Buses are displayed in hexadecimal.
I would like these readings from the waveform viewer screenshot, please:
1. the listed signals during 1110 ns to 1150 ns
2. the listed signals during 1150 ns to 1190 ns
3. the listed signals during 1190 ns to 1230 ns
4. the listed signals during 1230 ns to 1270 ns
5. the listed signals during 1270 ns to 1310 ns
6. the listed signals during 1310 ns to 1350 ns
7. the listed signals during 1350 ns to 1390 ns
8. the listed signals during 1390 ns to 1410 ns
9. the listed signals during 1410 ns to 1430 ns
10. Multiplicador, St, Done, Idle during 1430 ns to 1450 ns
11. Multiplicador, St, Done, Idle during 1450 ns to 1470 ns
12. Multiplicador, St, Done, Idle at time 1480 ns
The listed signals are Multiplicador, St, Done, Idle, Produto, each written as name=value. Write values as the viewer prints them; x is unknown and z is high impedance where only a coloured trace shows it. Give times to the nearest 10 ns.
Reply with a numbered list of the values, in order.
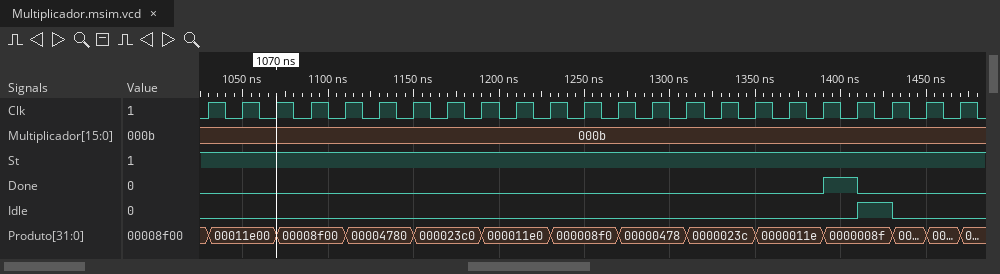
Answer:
1. Multiplicador=000b, St=1, Done=0, Idle=0, Produto=00004780
2. Multiplicador=000b, St=1, Done=0, Idle=0, Produto=000023c0
3. Multiplicador=000b, St=1, Done=0, Idle=0, Produto=000011e0
4. Multiplicador=000b, St=1, Done=0, Idle=0, Produto=000008f0
5. Multiplicador=000b, St=1, Done=0, Idle=0, Produto=00000478
6. Multiplicador=000b, St=1, Done=0, Idle=0, Produto=0000023c
7. Multiplicador=000b, St=1, Done=0, Idle=0, Produto=0000011e
8. Multiplicador=000b, St=1, Done=1, Idle=0, Produto=0000008f
9. Multiplicador=000b, St=1, Done=0, Idle=1, Produto=0000008f
10. Multiplicador=000b, St=1, Done=0, Idle=0
11. Multiplicador=000b, St=1, Done=0, Idle=0
12. Multiplicador=000b, St=1, Done=0, Idle=0
